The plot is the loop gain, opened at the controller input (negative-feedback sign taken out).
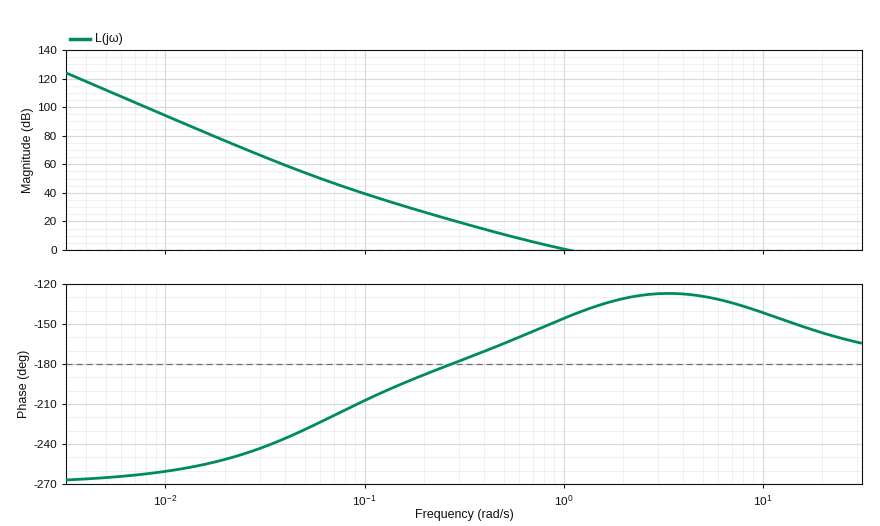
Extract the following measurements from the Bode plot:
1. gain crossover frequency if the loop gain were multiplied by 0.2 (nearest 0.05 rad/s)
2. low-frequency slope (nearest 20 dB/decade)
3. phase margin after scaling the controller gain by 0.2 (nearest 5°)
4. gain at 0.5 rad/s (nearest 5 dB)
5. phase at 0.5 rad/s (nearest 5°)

0.40 rad/s
-60 dB/decade
10°
10 dB
-165°
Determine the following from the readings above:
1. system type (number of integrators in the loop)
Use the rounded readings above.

3
